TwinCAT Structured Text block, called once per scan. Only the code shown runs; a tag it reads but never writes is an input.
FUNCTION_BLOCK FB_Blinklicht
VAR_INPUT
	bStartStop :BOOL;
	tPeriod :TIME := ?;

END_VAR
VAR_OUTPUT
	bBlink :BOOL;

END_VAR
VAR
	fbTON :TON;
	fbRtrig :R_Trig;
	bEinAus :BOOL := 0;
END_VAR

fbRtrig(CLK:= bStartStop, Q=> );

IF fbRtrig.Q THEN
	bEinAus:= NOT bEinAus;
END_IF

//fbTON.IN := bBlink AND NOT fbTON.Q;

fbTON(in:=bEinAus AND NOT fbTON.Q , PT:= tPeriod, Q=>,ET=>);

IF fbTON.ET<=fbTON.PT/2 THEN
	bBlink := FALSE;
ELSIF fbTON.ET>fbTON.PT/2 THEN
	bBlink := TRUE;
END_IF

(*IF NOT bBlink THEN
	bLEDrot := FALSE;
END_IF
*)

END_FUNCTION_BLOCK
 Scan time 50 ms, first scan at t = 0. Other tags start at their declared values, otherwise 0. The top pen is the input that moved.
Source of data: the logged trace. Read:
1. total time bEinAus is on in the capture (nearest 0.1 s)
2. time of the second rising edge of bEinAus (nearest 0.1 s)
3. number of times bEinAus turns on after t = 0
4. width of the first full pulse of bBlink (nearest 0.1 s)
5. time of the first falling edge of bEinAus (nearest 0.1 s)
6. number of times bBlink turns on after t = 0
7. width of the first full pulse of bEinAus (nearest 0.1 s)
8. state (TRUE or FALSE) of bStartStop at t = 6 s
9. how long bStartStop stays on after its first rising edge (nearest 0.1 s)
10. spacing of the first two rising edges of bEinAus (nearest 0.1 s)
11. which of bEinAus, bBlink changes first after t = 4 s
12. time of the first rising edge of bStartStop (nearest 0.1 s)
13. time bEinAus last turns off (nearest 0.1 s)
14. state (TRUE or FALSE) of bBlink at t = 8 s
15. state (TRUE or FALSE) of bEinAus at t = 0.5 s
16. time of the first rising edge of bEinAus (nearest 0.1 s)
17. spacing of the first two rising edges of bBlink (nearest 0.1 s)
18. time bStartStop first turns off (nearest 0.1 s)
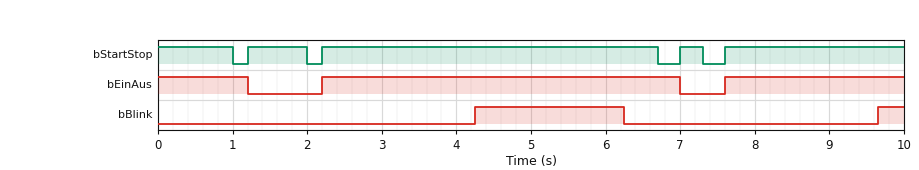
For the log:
8.4 s
7.6 s
2
2.0 s
1.2 s
2
4.8 s
TRUE
0.8 s
5.4 s
bBlink
1.2 s
7.0 s
FALSE
TRUE
2.2 s
5.4 s
1.0 s
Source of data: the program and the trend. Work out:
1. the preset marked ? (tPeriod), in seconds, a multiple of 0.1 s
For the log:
4.0 s
